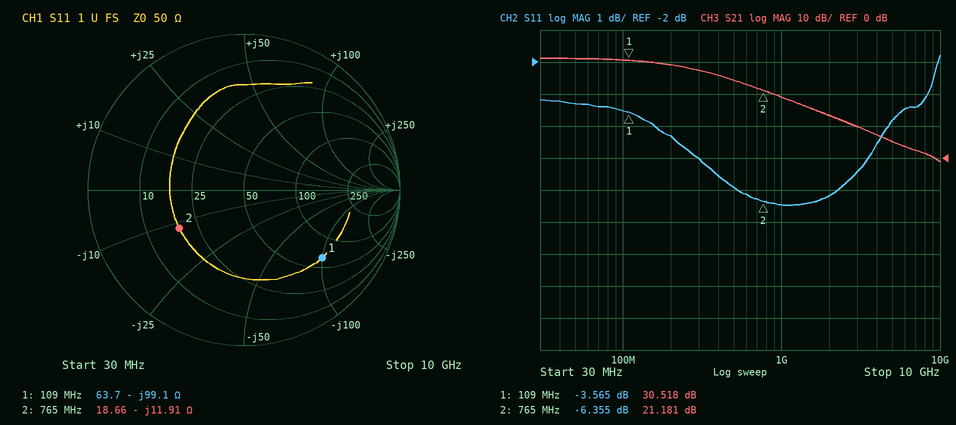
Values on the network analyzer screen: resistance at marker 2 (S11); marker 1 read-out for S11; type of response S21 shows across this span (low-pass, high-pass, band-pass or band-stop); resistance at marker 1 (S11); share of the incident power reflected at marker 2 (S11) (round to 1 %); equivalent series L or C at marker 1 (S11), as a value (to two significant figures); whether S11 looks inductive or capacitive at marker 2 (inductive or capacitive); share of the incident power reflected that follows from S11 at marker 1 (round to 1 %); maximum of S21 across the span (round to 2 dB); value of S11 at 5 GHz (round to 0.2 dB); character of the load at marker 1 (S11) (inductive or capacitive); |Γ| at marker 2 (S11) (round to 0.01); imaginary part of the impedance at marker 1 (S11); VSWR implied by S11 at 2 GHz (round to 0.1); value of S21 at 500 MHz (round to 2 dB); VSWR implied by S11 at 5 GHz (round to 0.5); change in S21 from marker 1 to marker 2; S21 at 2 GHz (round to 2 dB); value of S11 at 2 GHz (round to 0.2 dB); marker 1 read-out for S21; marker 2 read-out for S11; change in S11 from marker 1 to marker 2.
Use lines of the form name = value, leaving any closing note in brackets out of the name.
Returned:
resistance at marker 2 = 18.66 Ω
marker 1 read-out for S11 = -3.565 dB
type of response S21 shows across this span = low-pass
resistance at marker 1 = 63.7 Ω
share of the incident power reflected at marker 2 (S11) = 23 %
equivalent series L or C at marker 1 (S11), as a value = 15 pF
whether S11 looks inductive or capacitive at marker 2 = capacitive
share of the incident power reflected that follows from S11 at marker 1 = 44 %
maximum of S21 across the span = 32 dB
value of S11 at 5 GHz = -3.8 dB
character of the load at marker 1 (S11) = capacitive
|Γ| at marker 2 (S11) = 0.48
imaginary part of the impedance at marker 1 = -99.1 Ω
VSWR implied by S11 at 2 GHz = 2.9
value of S21 at 500 MHz = 24 dB
VSWR implied by S11 at 5 GHz = 4.5
change in S21 from marker 1 to marker 2 = -9.337 dB
S21 at 2 GHz = 14 dB
value of S11 at 2 GHz = -6.2 dB
marker 1 read-out for S21 = 30.518 dB
marker 2 read-out for S11 = -6.355 dB
change in S11 from marker 1 to marker 2 = -2.790 dB
